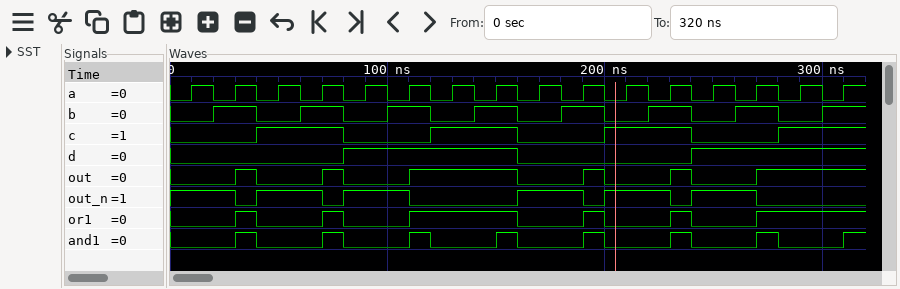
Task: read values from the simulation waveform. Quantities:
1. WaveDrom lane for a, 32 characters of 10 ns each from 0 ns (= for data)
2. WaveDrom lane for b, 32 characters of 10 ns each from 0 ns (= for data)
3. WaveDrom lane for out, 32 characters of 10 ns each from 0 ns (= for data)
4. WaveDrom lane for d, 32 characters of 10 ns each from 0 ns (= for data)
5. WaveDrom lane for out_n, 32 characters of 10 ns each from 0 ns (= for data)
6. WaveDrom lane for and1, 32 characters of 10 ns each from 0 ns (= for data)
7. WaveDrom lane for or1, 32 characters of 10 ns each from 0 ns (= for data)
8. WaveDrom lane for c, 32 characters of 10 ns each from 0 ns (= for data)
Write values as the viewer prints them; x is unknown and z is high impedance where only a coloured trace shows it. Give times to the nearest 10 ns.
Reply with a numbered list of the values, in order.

1. {name: 'a', wave: '01010101010101010101010101010101'}
2. {name: 'b', wave: '0.1.0.1.0.1.0.1.0.1.0.1.0.1.0.1.'}
3. {name: 'out', wave: '0..10..10..1....0..10..10..1....'}
4. {name: 'd', wave: '0.......1.......0.......1.......'}
5. {name: 'out_n', wave: '1..01..01..0....1..01..01..0....'}
6. {name: 'and1', wave: '0..10..10..10..10..10..10..10..1'}
7. {name: 'or1', wave: '0..10..10..1....0..10..10..1....'}
8. {name: 'c', wave: '0...1...0...1...0...1...0...1...'}
